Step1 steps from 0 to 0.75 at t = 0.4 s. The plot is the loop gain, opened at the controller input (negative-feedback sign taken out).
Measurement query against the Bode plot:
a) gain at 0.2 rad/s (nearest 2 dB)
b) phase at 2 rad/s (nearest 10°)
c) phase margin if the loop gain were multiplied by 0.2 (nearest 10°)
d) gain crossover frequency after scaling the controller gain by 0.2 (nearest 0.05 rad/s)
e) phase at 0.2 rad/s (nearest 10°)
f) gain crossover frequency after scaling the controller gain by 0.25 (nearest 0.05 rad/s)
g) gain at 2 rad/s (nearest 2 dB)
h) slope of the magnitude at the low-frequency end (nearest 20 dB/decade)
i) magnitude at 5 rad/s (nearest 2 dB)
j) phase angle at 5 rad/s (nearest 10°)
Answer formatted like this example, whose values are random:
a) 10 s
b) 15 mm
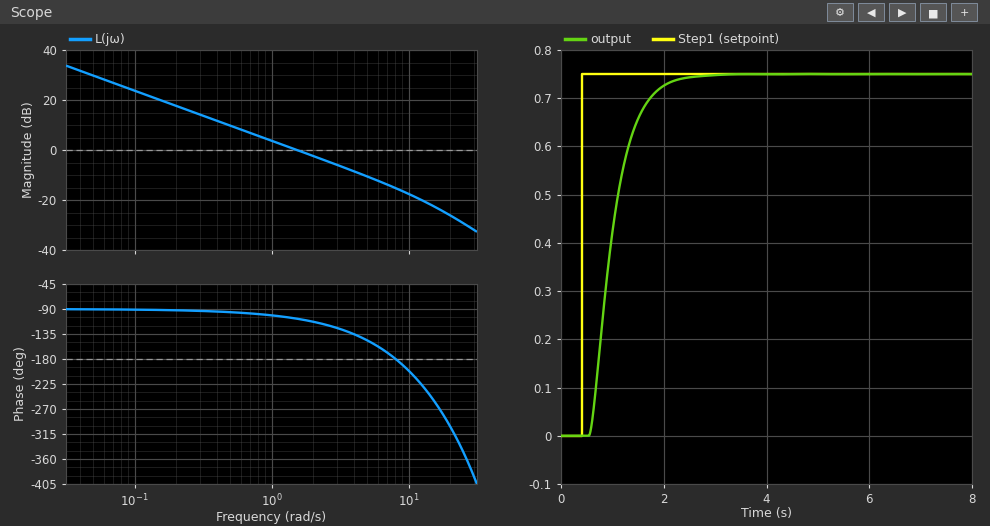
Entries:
a) 18 dB
b) -110°
c) 90°
d) 0.30 rad/s
e) -90°
f) 0.40 rad/s
g) -2 dB
h) -20 dB/decade
i) -10 dB
j) -150°
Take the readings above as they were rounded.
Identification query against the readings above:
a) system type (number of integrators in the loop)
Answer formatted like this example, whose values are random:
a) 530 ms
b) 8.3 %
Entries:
a) 1
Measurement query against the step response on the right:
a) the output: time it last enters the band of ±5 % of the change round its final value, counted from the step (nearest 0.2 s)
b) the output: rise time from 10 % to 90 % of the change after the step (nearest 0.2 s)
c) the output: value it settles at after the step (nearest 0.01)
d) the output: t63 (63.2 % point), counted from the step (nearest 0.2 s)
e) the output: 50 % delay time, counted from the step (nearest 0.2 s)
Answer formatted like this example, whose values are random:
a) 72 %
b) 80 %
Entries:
a) 1.4 s
b) 1.0 s
c) 0.75
d) 0.6 s
e) 0.6 s
